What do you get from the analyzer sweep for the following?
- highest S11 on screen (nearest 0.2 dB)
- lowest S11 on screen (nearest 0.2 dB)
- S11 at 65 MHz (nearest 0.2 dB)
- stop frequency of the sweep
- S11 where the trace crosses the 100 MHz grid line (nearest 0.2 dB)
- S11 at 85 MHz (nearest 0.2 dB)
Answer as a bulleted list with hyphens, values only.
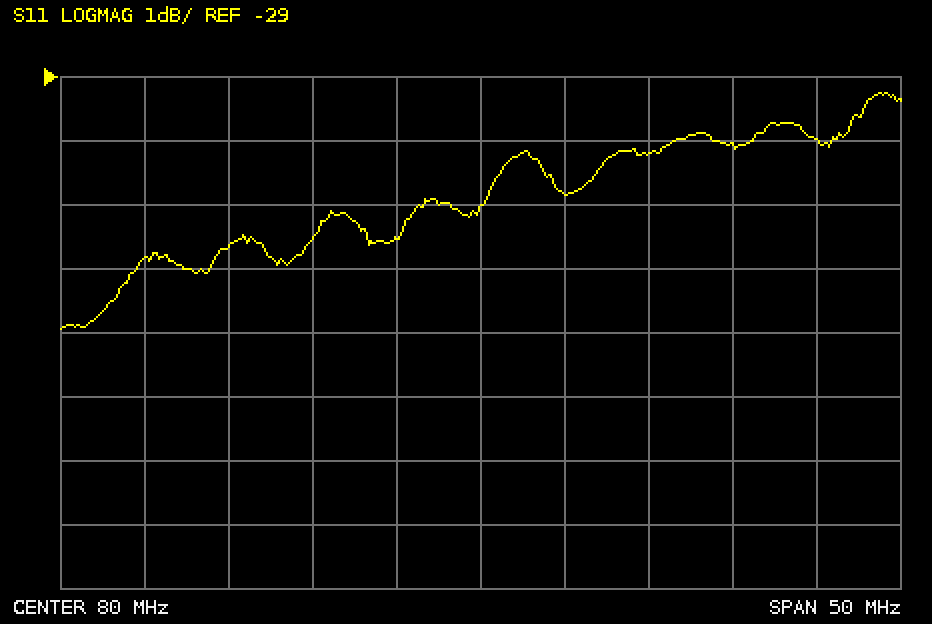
- -29.2 dB
- -33.0 dB
- -31.6 dB
- 105 MHz
- -30.0 dB
- -30.8 dB
